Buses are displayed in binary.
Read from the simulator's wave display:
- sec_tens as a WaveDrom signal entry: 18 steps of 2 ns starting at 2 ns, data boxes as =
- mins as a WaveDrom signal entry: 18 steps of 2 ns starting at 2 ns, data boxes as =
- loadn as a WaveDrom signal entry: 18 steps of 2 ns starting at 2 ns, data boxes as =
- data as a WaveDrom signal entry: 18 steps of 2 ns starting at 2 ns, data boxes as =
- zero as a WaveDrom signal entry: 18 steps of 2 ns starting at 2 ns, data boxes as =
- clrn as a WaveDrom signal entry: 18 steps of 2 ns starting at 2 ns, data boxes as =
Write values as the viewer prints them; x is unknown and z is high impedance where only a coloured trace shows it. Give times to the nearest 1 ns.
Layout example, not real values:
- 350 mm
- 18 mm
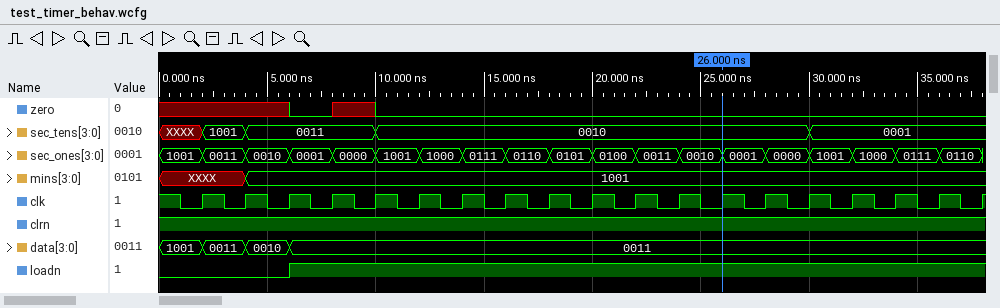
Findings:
- {name: 'sec_tens', wave: '==..=.........=...', data: '1001 0011 0010 0001'}
- {name: 'mins', wave: 'x=................', data: '1001'}
- {name: 'loadn', wave: '0.1...............'}
- {name: 'data', wave: '===...............', data: '0011 0010 0011'}
- {name: 'zero', wave: 'x.0x0.............'}
- {name: 'clrn', wave: '1.................'}
